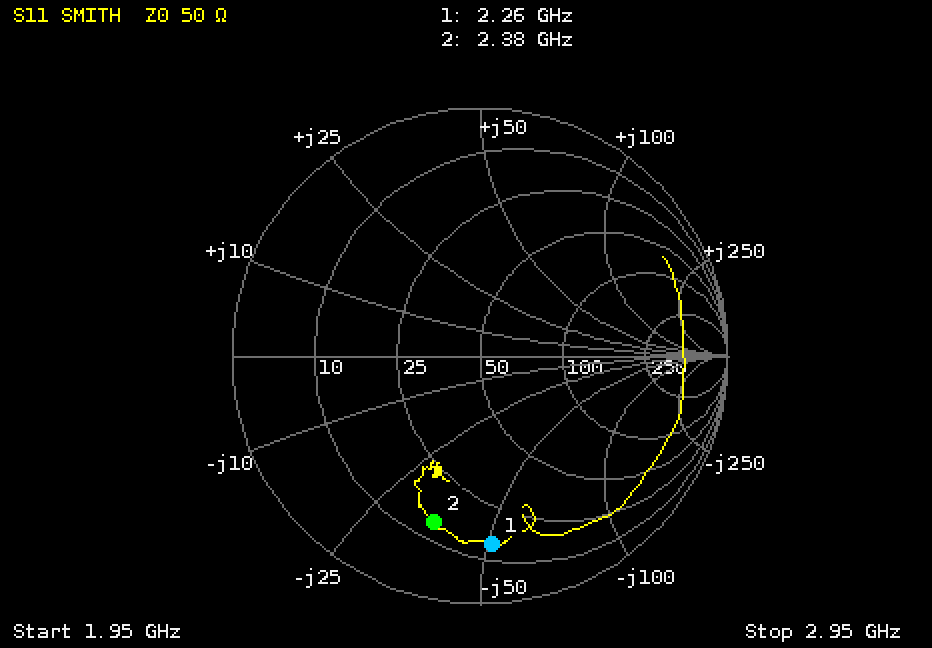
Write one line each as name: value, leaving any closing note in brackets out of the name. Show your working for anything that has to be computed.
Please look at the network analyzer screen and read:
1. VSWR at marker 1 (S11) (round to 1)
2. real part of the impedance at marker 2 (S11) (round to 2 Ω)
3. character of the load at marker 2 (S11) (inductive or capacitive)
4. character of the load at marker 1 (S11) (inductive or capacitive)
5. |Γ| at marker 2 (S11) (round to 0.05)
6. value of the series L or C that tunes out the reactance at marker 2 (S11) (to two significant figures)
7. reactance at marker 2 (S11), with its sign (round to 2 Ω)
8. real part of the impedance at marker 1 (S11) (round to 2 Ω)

VSWR at marker 1 (S11): 7
real part of the impedance at marker 2 (S11): 14 Ω
character of the load at marker 2 (S11): capacitive
character of the load at marker 1 (S11): capacitive
|Γ| at marker 2 (S11): 0.70
value of the series L or C that tunes out the reactance at marker 2 (S11): L = 36 Ω/(2π × 2.38 GHz) ≈ 2.4 nH
reactance at marker 2 (S11), with its sign: -36 Ω
real part of the impedance at marker 1 (S11): 14 Ω
